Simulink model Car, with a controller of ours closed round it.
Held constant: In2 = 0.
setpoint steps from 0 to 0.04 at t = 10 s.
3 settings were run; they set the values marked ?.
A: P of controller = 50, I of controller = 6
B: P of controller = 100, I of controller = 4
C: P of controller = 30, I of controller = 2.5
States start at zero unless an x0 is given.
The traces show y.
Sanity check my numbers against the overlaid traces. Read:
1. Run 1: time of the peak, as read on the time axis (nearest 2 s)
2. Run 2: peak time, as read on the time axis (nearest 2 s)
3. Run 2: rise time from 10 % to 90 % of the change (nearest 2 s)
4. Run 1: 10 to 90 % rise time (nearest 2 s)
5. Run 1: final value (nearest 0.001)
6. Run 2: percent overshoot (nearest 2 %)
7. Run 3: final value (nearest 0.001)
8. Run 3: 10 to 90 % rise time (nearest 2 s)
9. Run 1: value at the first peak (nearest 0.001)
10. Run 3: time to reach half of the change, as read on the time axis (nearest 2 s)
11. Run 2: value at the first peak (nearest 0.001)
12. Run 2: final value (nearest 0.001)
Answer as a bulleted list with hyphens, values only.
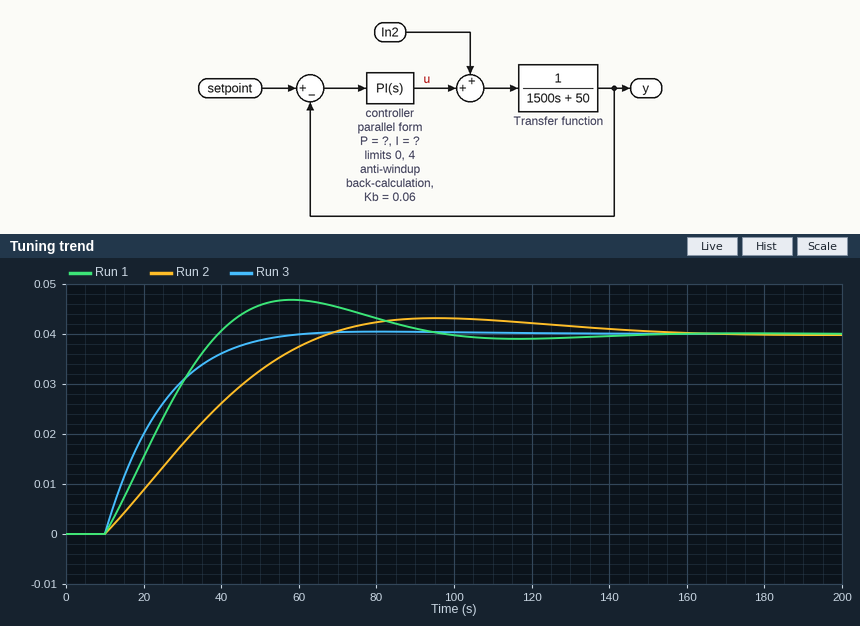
- 58 s
- 96 s
- 42 s
- 22 s
- 0.040
- 8 %
- 0.040
- 28 s
- 0.047
- 20 s
- 0.043
- 0.040
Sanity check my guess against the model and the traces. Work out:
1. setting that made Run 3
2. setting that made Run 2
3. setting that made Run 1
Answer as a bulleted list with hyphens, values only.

- B
- C
- A
